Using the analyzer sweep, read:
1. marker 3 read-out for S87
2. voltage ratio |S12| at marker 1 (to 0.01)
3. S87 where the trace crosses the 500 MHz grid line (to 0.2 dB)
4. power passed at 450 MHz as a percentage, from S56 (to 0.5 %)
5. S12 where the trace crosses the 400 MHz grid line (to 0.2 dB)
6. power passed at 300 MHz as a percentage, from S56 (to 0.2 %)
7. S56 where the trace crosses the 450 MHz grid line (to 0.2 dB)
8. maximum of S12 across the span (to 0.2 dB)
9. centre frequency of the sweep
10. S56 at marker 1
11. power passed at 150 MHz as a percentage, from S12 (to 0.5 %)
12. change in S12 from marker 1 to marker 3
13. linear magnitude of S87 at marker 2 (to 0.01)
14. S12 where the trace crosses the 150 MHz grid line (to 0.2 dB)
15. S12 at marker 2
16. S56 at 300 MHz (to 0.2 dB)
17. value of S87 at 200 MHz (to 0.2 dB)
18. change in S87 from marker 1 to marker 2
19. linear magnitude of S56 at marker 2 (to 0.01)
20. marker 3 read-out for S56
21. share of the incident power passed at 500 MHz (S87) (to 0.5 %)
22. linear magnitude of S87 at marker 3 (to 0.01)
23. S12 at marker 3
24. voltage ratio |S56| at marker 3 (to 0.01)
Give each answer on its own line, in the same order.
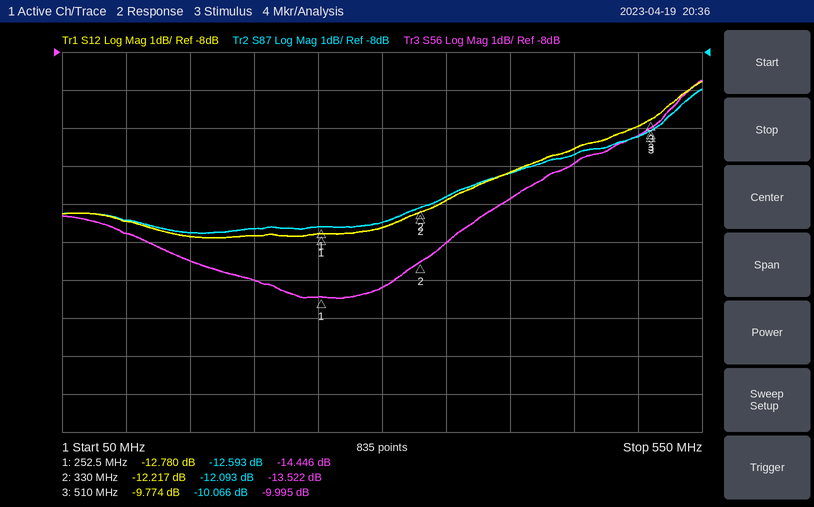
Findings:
-10.066 dB
0.23
-10.2 dB
8.0 %
-11.2 dB
3.8 %
-11.0 dB
-8.8 dB
300 MHz
-14.446 dB
5.0 %
3.006 dB
0.25
-12.8 dB
-12.217 dB
-14.2 dB
-12.6 dB
0.500 dB
0.21
-9.995 dB
9.5 %
0.31
-9.774 dB
0.32
